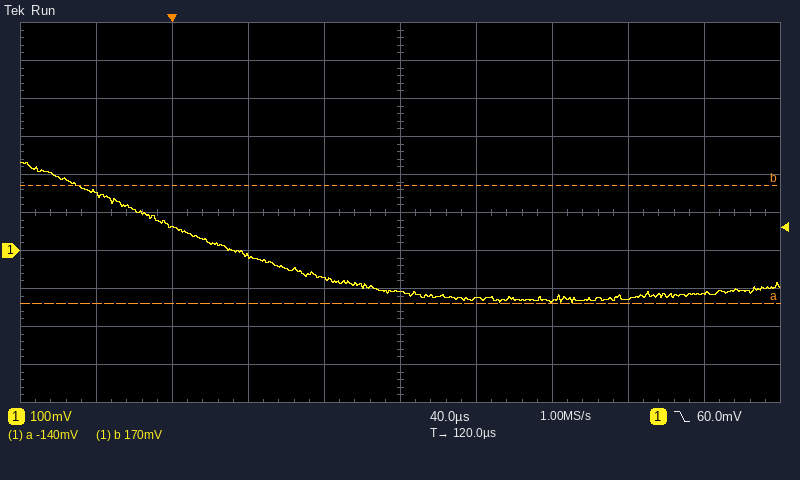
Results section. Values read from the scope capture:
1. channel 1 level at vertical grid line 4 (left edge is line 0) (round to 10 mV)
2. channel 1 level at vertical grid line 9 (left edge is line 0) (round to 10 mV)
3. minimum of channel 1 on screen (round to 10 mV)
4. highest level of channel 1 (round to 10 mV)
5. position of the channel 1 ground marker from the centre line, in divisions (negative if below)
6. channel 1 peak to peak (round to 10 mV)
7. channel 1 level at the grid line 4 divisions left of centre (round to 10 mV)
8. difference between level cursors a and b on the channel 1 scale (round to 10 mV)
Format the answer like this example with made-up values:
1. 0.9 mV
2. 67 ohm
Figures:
1. -70 mV
2. -110 mV
3. -140 mV
4. 230 mV
5. -1.0 div
6. 370 mV
7. 150 mV
8. 310 mV
